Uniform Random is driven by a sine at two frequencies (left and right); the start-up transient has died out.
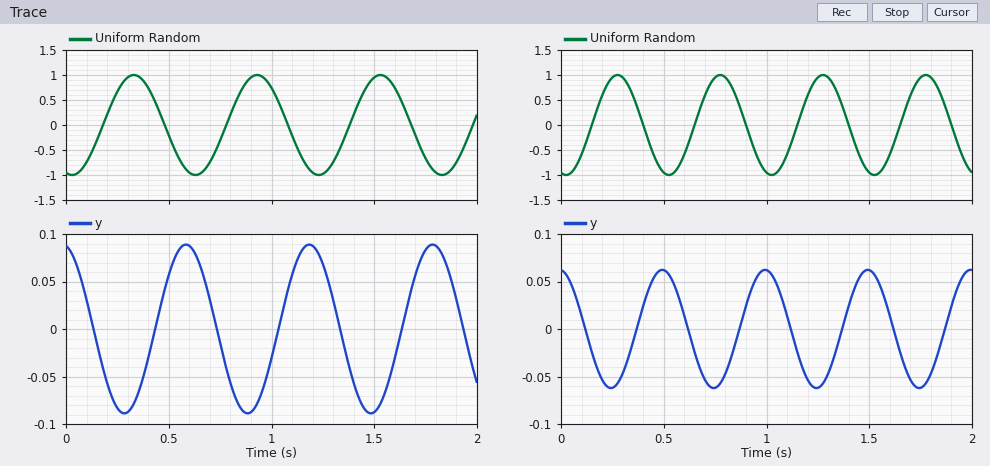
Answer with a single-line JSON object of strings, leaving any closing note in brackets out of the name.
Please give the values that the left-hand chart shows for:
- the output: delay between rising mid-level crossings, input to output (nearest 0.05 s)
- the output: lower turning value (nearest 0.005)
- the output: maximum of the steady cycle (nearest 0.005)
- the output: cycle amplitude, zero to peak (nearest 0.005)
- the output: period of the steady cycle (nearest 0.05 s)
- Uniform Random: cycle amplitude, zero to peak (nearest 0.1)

{"the output: delay between rising mid-level crossings, input to output": "0.25 s", "the output: lower turning value": "-0.090", "the output: maximum of the steady cycle": "0.090", "the output: cycle amplitude, zero to peak": "0.090", "the output: period of the steady cycle": "0.60 s", "Uniform Random: cycle amplitude, zero to peak": "1.0"}
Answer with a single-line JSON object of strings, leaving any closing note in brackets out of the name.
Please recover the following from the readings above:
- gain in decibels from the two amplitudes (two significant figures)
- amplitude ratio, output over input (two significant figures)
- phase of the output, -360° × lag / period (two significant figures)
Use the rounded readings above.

{"gain in decibels from the two amplitudes": "-21 dB", "amplitude ratio, output over input": "0.090", "phase of the output, -360° × lag / period": "-150°"}
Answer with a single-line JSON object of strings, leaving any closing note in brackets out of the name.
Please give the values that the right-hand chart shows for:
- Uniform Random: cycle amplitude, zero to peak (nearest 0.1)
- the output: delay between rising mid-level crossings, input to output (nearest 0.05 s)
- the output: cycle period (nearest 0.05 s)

{"Uniform Random: cycle amplitude, zero to peak": "1.0", "the output: delay between rising mid-level crossings, input to output": "0.20 s", "the output: cycle period": "0.50 s"}
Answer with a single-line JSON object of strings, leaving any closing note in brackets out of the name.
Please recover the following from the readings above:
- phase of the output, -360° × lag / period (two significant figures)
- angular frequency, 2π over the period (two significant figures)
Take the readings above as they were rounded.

{"phase of the output, -360° × lag / period": "-140°", "angular frequency, 2π over the period": "13 rad/s"}
